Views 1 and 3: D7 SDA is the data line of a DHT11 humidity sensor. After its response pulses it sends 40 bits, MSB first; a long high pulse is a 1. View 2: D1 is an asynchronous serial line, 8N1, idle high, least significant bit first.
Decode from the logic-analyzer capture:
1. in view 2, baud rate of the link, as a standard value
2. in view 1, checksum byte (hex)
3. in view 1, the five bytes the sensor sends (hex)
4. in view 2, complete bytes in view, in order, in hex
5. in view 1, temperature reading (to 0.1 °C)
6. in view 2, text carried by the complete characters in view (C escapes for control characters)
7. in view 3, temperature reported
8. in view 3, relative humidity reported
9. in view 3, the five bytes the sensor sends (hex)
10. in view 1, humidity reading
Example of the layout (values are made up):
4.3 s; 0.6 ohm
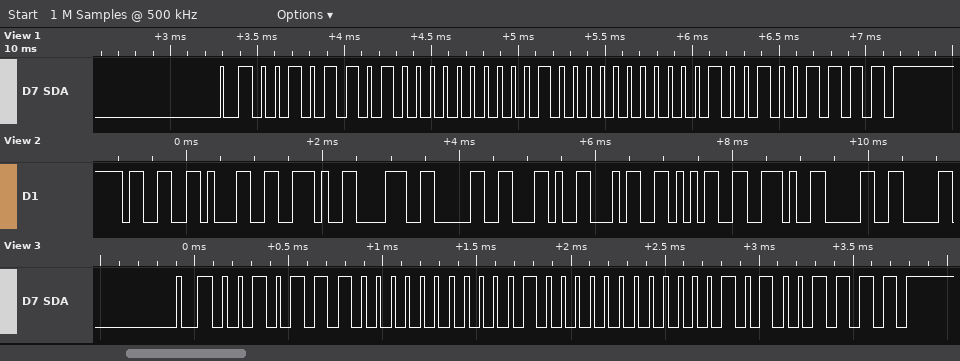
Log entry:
9600 baud; 0x4F; 2D 00 20 02 4F; 33 31 2E 38 30 2C 34 35 2E 30; 32.2 °C; "31.80,45.0"; 32.1 °C; 46 %; 2E 00 20 01 4F; 45 %
